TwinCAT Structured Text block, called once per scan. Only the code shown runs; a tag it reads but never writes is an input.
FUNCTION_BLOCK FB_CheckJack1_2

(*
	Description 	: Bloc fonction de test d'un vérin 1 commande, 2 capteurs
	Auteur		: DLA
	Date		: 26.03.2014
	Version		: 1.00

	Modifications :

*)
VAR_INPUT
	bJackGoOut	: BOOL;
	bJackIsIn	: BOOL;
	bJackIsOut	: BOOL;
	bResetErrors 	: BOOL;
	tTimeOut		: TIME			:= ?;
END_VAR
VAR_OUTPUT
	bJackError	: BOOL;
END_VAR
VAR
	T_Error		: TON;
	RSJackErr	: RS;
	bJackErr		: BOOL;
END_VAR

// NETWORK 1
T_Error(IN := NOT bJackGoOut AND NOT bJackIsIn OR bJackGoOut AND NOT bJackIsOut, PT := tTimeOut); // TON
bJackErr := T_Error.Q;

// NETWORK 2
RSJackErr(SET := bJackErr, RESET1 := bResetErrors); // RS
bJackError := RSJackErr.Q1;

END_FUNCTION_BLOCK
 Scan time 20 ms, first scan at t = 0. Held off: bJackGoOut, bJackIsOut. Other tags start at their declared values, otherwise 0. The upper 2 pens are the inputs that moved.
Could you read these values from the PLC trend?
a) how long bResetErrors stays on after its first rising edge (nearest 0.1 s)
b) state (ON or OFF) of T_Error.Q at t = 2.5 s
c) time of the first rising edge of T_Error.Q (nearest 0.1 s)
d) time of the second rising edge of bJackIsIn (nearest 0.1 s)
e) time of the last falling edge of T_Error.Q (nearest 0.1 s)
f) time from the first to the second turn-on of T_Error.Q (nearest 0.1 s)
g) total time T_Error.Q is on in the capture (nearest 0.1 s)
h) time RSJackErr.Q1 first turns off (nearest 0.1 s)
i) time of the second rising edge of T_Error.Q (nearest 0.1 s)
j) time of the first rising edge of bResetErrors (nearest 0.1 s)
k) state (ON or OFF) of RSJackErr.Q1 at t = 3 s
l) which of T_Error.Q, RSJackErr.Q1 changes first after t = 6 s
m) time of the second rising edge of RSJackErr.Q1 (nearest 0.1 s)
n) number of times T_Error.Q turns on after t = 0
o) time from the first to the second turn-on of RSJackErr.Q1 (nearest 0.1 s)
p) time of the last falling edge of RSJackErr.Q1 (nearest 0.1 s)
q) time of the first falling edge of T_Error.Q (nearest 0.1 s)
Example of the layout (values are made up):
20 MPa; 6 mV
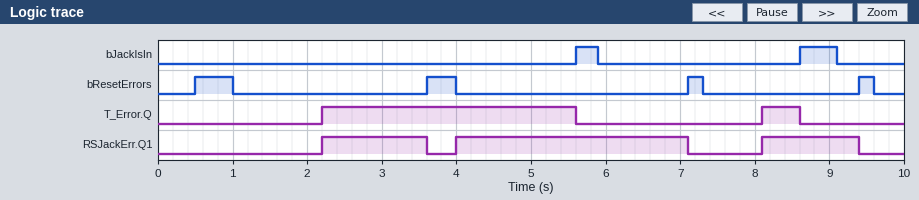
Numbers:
0.5 s; ON; 2.2 s; 8.6 s; 8.6 s; 5.9 s; 3.9 s; 3.6 s; 8.1 s; 0.5 s; ON; RSJackErr.Q1; 4.0 s; 2; 1.8 s; 9.4 s; 5.6 s
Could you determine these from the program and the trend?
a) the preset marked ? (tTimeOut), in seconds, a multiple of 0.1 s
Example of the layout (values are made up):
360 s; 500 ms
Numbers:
2.2 s
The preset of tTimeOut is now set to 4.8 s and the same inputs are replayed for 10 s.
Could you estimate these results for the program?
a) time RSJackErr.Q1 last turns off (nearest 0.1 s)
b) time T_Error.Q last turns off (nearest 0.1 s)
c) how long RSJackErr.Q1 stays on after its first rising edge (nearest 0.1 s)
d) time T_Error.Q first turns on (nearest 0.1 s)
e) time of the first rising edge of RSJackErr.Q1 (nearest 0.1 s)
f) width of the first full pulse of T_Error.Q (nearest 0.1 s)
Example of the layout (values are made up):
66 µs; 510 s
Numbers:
7.1 s; 5.6 s; 2.3 s; 4.8 s; 4.8 s; 0.8 s
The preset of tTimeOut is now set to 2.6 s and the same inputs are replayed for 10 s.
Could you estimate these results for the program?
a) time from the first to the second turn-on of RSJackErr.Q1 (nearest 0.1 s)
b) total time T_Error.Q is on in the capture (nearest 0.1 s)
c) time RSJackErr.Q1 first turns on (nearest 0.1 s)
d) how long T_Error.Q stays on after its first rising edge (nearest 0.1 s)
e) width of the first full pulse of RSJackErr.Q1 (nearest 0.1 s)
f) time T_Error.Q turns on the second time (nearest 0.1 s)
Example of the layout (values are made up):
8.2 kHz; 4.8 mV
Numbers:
1.4 s; 3.1 s; 2.6 s; 3.0 s; 1.0 s; 8.5 s
